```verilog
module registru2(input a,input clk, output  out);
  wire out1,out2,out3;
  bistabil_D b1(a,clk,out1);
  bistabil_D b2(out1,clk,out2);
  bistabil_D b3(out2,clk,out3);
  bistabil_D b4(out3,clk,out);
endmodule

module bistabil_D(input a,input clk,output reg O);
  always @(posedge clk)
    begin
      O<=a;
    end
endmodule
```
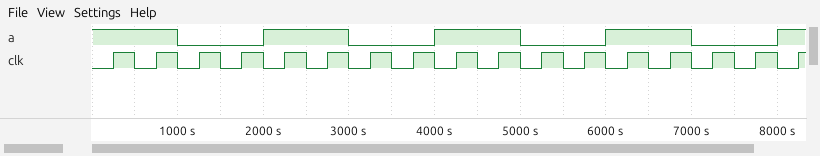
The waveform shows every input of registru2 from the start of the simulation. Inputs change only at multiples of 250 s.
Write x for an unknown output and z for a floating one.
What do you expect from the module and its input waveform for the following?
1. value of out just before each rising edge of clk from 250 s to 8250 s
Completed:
x x x x 1 1 0 0 1 1 0 0 1 1 0 0 1
